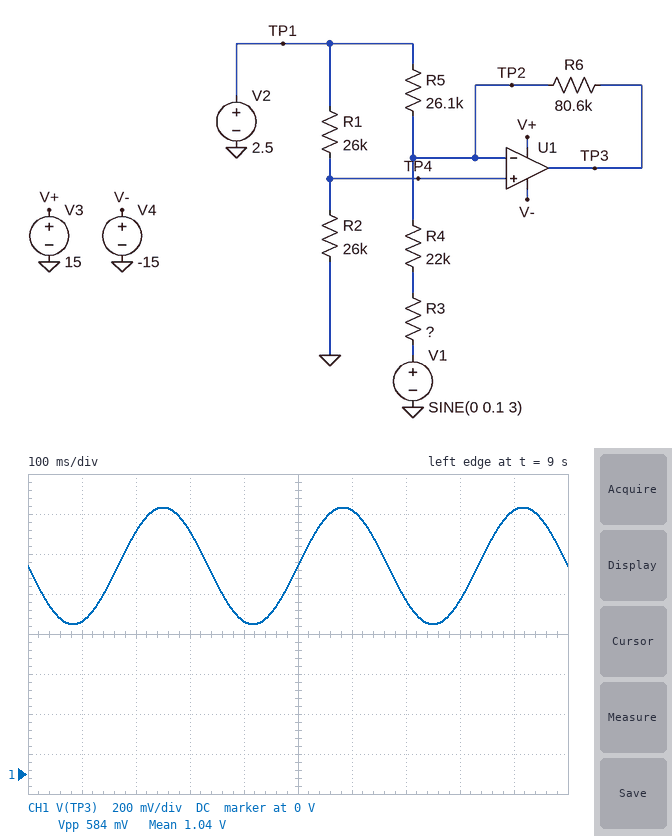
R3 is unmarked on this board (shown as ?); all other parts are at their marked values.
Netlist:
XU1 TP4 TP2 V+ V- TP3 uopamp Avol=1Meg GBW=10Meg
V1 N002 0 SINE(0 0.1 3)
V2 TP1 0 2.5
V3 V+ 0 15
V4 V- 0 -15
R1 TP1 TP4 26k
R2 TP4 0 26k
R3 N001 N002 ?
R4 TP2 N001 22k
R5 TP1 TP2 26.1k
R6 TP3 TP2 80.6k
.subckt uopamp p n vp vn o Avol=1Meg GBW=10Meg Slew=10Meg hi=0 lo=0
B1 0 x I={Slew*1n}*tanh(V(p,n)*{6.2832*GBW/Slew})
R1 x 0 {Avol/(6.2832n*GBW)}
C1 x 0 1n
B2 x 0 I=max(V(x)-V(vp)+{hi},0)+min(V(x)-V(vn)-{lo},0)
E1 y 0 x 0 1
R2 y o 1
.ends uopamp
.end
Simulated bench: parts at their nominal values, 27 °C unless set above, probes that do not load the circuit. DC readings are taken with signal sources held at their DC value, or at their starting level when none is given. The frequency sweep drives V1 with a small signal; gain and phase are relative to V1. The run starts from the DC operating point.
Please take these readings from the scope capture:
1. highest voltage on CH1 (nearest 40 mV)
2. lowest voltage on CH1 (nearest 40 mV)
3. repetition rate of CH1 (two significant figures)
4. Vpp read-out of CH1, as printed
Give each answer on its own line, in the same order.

1.32 V
760 mV
3.0 Hz
584 mV
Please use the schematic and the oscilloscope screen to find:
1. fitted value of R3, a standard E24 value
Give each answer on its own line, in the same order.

5.6 kΩ
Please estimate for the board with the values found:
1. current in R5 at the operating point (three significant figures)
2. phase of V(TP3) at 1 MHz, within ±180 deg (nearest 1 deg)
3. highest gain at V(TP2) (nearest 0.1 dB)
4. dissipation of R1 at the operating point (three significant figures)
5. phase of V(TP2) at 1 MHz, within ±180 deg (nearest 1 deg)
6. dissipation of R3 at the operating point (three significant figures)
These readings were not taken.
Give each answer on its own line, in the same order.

47.9 µA
145 deg
-7.6 dB
60.1 µW
55 deg
11.5 µW
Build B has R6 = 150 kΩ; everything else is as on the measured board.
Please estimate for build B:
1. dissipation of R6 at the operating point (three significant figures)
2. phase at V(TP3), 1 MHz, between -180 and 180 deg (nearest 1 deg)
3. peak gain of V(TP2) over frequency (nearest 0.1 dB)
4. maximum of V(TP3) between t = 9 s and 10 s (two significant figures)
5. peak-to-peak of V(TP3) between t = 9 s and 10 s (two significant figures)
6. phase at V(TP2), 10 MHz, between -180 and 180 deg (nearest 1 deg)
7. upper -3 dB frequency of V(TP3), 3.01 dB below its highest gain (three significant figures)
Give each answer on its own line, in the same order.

1.02 µW
129 deg
-7.0 dB
1.4 V
1.1 V
5 deg
821 kHz
